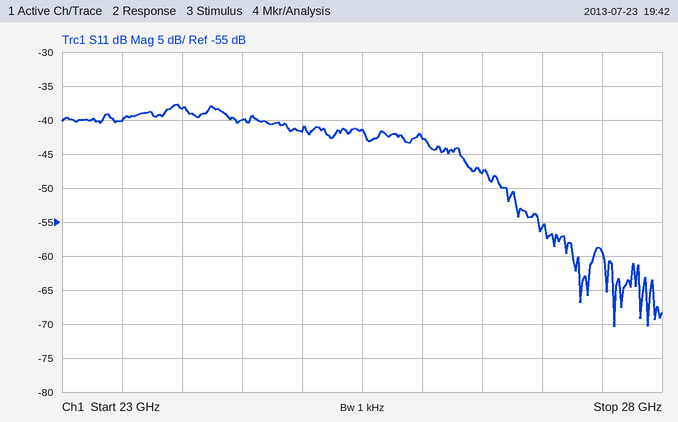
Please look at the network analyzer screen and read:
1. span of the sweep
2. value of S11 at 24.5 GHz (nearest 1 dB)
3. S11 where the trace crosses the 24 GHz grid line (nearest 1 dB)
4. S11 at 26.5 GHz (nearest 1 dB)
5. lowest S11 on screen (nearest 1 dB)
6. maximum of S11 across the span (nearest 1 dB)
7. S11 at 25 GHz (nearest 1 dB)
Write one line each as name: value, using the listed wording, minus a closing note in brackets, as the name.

span of the sweep: 5 GHz
value of S11 at 24.5 GHz: -40 dB
S11 where the trace crosses the 24 GHz grid line: -38 dB
S11 at 26.5 GHz: -48 dB
lowest S11 on screen: -70 dB
maximum of S11 across the span: -38 dB
S11 at 25 GHz: -42 dB
